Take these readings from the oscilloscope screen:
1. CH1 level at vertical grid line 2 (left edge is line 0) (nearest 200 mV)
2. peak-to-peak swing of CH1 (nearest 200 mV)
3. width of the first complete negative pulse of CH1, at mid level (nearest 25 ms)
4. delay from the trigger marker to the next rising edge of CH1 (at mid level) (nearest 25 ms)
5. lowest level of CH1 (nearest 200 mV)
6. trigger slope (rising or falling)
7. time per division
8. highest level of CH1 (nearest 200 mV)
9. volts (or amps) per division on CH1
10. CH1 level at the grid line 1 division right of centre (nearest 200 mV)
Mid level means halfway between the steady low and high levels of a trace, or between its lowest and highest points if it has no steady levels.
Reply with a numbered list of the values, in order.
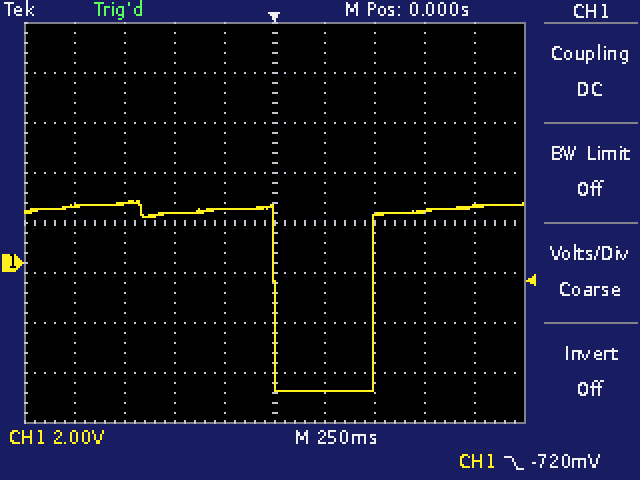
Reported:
1. 2.4 V
2. 7.6 V
3. 500 ms
4. 500 ms
5. -5.2 V
6. falling
7. 250 ms
8. 2.4 V
9. 2 V
10. -5.2 V
